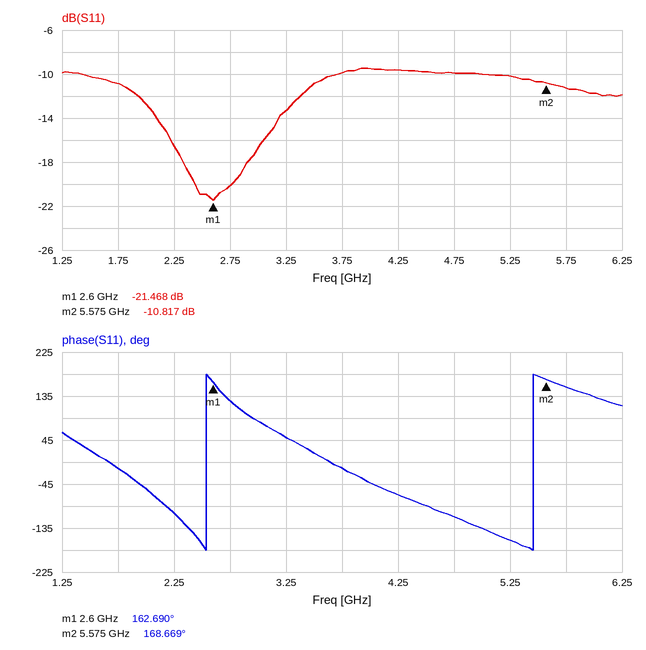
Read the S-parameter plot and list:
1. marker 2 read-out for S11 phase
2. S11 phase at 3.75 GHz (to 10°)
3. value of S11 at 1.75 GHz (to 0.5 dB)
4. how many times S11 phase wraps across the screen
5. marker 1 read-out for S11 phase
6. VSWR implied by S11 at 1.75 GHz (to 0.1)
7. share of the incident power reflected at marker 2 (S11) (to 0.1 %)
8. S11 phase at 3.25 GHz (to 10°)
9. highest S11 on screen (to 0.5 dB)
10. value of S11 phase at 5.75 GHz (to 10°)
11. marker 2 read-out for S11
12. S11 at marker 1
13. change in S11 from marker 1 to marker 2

168.669°
-10°
-11.0 dB
2
162.690°
1.8
8.3 %
50°
-9.5 dB
150°
-10.817 dB
-21.468 dB
10.651 dB
